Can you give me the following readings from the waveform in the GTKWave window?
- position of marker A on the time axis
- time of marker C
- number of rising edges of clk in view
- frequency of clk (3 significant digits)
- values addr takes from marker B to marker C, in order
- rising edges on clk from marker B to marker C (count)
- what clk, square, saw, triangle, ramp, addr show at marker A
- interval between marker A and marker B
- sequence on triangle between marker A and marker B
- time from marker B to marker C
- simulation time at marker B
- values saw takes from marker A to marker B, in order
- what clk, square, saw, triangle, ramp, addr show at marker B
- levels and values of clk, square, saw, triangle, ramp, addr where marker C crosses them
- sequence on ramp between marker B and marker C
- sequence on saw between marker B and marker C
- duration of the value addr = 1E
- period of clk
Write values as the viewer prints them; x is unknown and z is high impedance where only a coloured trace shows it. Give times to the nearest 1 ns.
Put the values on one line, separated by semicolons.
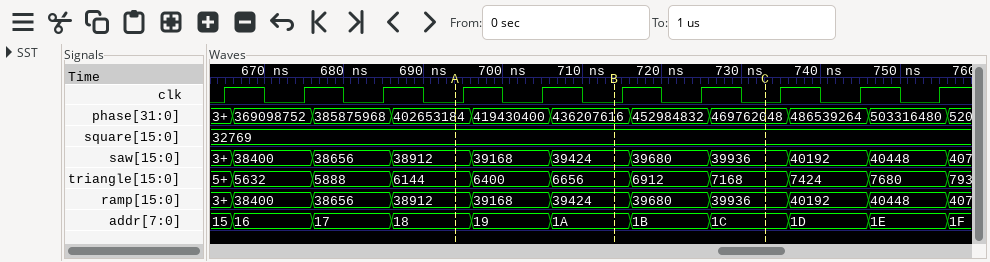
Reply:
694 ns; 733 ns; 10; 100 MHz; 1A, 1B, 1C; 2; clk=0, square=32769, saw=38912, triangle=6144, ramp=38912, addr=18; 20 ns; 6144, 6400, 6656; 19 ns; 714 ns; 38912, 39168, 39424; clk=0, square=32769, saw=39424, triangle=6656, ramp=39424, addr=1A; clk=0, square=32769, saw=39936, triangle=7168, ramp=39936, addr=1C; 39424, 39680, 39936; 39424, 39680, 39936; 10 ns; 10 ns
